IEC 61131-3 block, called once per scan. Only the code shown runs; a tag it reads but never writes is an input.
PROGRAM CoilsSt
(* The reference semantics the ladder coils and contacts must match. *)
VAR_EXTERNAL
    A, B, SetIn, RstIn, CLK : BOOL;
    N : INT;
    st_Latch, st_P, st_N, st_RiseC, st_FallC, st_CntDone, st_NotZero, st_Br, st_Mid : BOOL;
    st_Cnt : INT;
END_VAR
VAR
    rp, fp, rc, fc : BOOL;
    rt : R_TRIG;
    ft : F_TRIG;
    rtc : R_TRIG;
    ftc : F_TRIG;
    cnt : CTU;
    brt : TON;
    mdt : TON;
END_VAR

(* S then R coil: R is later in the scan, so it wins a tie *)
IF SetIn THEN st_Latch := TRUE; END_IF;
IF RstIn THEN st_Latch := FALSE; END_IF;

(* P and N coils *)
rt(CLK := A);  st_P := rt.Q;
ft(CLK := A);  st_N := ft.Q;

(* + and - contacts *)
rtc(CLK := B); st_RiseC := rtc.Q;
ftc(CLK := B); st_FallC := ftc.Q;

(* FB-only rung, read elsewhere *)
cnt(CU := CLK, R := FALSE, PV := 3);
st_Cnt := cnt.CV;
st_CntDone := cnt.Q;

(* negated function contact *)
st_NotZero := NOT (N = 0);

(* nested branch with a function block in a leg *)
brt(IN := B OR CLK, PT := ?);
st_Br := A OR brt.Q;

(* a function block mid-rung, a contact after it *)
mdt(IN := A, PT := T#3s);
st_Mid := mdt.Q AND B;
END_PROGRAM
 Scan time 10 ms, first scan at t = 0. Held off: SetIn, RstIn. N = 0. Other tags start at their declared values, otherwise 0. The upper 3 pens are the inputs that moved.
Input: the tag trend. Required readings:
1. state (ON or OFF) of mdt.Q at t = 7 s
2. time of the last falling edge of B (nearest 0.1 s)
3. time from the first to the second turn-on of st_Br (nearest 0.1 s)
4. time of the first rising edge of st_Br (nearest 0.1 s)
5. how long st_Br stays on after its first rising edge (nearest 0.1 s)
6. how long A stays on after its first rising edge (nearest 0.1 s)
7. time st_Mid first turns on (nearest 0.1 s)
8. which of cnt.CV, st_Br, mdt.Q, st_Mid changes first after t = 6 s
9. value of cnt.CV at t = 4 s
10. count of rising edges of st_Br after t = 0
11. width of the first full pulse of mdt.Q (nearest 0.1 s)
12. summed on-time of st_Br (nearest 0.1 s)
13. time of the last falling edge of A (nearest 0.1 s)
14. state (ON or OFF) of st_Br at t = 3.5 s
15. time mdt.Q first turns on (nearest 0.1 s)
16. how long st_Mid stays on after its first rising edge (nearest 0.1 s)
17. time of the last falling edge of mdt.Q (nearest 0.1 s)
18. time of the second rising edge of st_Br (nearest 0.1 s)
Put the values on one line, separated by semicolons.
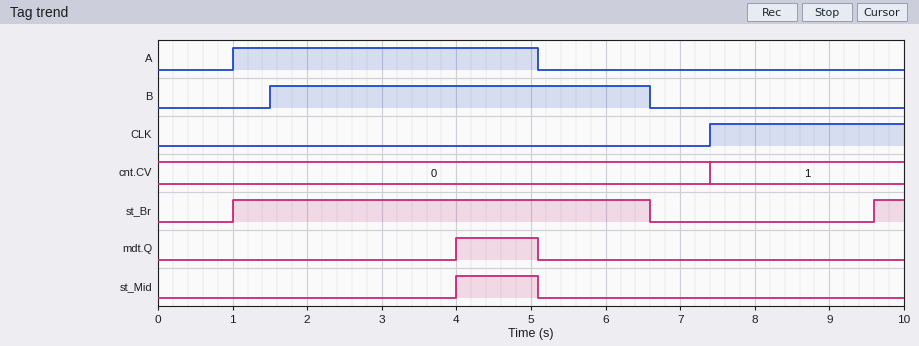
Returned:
OFF; 6.6 s; 8.6 s; 1.0 s; 5.6 s; 4.1 s; 4.0 s; st_Br; 0; 2; 1.1 s; 6.0 s; 5.1 s; ON; 4.0 s; 1.1 s; 5.1 s; 9.6 s
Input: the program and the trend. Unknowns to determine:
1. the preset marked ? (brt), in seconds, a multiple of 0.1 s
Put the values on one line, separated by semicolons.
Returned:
2.2 s
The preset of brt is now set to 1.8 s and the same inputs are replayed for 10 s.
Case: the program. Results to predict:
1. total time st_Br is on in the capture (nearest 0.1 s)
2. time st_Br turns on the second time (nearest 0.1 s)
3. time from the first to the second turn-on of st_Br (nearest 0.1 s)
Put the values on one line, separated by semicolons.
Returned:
6.4 s; 9.2 s; 8.2 s
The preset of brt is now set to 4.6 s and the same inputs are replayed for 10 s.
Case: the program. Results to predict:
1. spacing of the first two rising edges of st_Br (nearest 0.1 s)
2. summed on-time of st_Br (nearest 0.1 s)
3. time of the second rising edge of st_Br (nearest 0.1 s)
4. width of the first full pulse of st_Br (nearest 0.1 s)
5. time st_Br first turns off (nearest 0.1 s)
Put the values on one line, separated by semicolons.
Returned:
5.1 s; 4.6 s; 6.1 s; 4.1 s; 5.1 s
